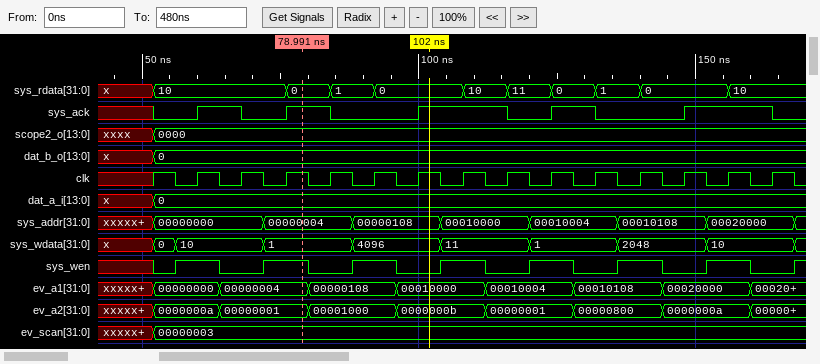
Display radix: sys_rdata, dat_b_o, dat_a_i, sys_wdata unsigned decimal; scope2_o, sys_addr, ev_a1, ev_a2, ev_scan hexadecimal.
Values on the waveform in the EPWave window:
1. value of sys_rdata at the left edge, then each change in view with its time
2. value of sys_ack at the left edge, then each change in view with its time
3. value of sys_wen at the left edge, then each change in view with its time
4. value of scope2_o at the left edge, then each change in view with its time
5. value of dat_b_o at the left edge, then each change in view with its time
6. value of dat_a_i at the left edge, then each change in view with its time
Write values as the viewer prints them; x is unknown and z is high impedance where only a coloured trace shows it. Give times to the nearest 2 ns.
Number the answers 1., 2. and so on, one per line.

1. x, 10 at 52 ns, 0 at 76 ns, 1 at 84 ns, 0 at 92 ns, 10 at 108 ns, 11 at 116 ns, 0 at 124 ns, 1 at 132 ns, 0 at 140 ns, 10 at 156 ns
2. x, 0 at 52 ns, 1 at 60 ns, 0 at 68 ns, 1 at 76 ns, 0 at 84 ns, 1 at 100 ns, 0 at 116 ns, 1 at 124 ns, 0 at 132 ns, 1 at 148 ns, 0 at 164 ns
3. x, 0 at 52 ns, 1 at 56 ns, 0 at 64 ns, 1 at 72 ns, 0 at 80 ns, 1 at 88 ns, 0 at 96 ns, 1 at 104 ns, 0 at 112 ns, 1 at 120 ns, 0 at 128 ns, 1 at 136 ns, 0 at 144 ns, 1 at 152 ns, 0 at 160 ns, 1 at 168 ns
4. xxxx, 0000 at 52 ns
5. x, 0 at 52 ns
6. x, 0 at 52 ns
